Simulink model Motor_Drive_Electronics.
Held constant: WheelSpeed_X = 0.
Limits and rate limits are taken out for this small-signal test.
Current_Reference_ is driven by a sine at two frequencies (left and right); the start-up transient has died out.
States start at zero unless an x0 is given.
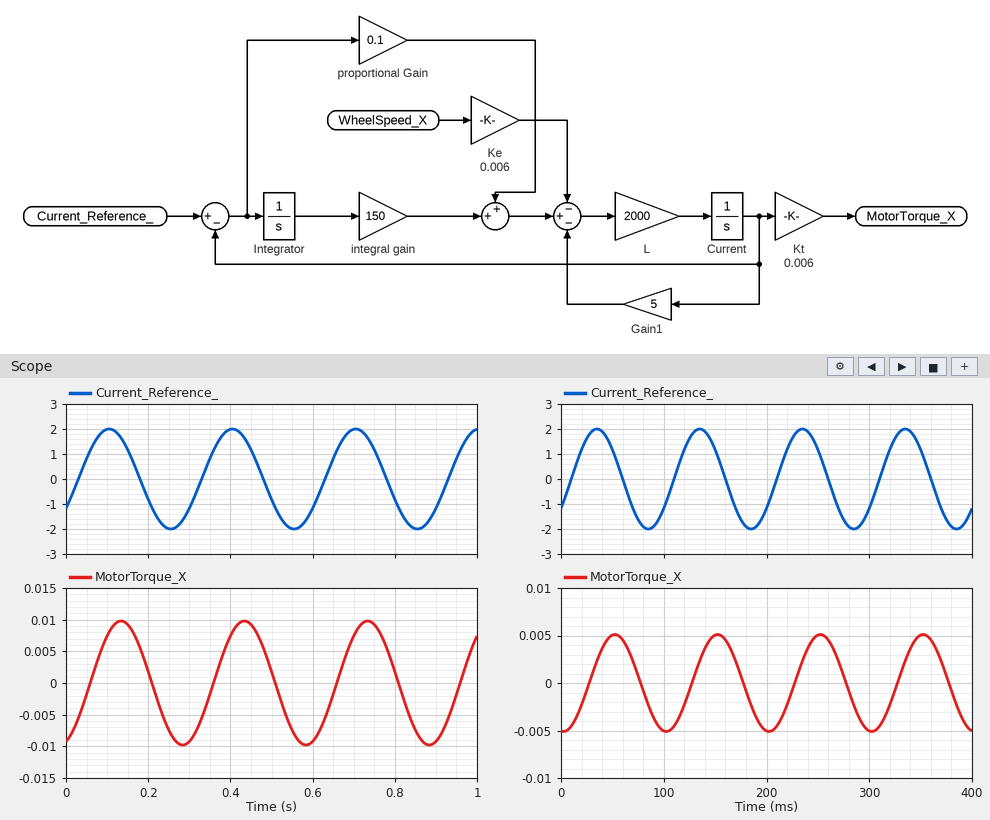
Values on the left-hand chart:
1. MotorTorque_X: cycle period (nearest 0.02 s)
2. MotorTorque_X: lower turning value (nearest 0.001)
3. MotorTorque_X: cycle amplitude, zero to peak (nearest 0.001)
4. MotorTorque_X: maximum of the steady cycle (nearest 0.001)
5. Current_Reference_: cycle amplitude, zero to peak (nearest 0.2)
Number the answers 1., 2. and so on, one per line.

1. 0.30 s
2. -0.010
3. 0.010
4. 0.010
5. 2.0
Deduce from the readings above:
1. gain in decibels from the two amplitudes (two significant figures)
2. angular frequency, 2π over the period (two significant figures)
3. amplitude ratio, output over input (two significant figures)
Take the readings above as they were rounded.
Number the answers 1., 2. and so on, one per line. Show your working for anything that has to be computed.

1. 20 log10(0.01 / 2) = -46 dB
2. 2π / 0.3 = 21 rad/s
3. 0.01 / 2 = 0.0050
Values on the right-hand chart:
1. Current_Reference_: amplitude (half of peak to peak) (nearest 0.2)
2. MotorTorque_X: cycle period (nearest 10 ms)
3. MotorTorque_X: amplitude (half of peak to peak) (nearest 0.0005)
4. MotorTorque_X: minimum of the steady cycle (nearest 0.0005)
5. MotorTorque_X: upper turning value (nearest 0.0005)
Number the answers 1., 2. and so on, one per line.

1. 2.0
2. 100 ms
3. 0.0050
4. -0.0050
5. 0.0050
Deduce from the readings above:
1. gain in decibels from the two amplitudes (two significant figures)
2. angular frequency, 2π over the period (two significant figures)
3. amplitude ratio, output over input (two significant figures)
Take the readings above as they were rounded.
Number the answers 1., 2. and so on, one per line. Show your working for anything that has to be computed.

1. 20 log10(0.005 / 2) = -52 dB
2. 2π / 100 = 0.063 rad/ms
3. 0.005 / 2 = 0.0025
